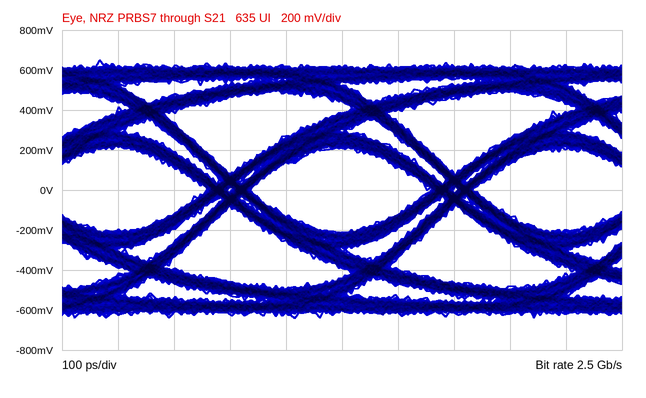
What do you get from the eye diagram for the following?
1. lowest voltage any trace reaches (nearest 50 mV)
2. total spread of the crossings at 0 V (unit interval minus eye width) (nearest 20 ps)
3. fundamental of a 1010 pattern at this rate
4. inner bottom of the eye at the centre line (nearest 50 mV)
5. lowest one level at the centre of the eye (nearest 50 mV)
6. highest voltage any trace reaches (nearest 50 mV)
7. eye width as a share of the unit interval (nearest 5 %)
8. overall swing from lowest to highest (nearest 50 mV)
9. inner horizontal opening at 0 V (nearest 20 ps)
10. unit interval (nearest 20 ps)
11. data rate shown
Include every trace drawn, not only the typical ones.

-650 mV
80 ps
1.25 GHz
-200 mV
200 mV
650 mV
80 %
1.30 V
320 ps
400 ps
2.5 Gb/s
